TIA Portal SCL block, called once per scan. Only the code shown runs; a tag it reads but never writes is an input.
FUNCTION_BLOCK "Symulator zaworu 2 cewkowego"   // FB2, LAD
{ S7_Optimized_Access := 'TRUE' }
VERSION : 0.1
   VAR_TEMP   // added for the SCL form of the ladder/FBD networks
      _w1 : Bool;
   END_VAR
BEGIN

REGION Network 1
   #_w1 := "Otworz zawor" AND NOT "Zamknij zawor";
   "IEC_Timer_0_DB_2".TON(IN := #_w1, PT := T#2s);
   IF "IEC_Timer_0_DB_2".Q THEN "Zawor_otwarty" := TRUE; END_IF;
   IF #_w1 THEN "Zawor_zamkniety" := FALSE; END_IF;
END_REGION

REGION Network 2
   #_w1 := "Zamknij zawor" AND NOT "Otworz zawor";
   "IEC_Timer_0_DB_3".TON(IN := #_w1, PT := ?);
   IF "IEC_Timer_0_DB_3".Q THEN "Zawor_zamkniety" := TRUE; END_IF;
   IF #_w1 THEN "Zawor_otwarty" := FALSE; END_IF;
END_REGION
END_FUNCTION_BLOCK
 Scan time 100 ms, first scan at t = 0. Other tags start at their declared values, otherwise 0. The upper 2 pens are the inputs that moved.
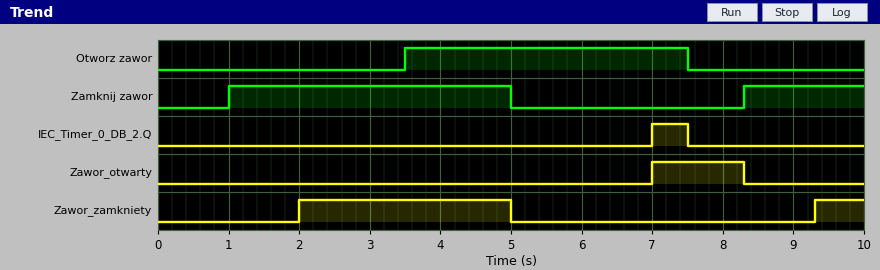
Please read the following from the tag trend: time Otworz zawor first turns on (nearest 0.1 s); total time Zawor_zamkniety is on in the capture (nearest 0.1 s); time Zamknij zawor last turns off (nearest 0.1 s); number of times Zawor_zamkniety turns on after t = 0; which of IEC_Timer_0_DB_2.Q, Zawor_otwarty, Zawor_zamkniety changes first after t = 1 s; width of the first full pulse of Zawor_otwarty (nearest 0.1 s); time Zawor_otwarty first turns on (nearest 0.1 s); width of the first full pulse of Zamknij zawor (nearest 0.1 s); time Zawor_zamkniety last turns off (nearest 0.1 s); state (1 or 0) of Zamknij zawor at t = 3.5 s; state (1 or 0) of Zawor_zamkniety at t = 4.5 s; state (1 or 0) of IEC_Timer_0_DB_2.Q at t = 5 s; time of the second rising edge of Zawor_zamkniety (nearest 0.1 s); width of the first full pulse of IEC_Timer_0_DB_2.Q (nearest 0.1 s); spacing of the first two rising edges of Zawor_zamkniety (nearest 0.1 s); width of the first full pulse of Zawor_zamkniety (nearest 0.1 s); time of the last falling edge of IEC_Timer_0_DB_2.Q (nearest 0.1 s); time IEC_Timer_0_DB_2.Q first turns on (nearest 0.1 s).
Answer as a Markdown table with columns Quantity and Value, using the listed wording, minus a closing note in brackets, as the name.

| Quantity | Value |
|---|---|
| time Otworz zawor first turns on | 3.5 s |
| total time Zawor_zamkniety is on in the capture | 3.7 s |
| time Zamknij zawor last turns off | 5.0 s |
| number of times Zawor_zamkniety turns on after t = 0 | 2 |
| which of IEC_Timer_0_DB_2.Q, Zawor_otwarty, Zawor_zamkniety changes first after t = 1 s | Zawor_zamkniety |
| width of the first full pulse of Zawor_otwarty | 1.3 s |
| time Zawor_otwarty first turns on | 7.0 s |
| width of the first full pulse of Zamknij zawor | 4.0 s |
| time Zawor_zamkniety last turns off | 5.0 s |
| state (1 or 0) of Zamknij zawor at t = 3.5 s | 1 |
| state (1 or 0) of Zawor_zamkniety at t = 4.5 s | 1 |
| state (1 or 0) of IEC_Timer_0_DB_2.Q at t = 5 s | 0 |
| time of the second rising edge of Zawor_zamkniety | 9.3 s |
| width of the first full pulse of IEC_Timer_0_DB_2.Q | 0.5 s |
| spacing of the first two rising edges of Zawor_zamkniety | 7.3 s |
| width of the first full pulse of Zawor_zamkniety | 3.0 s |
| time of the last falling edge of IEC_Timer_0_DB_2.Q | 7.5 s |
| time IEC_Timer_0_DB_2.Q first turns on | 7.0 s |
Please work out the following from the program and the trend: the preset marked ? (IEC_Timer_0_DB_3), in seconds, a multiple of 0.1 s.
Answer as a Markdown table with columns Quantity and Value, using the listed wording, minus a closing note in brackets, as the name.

| Quantity | Value |
|---|---|
| the preset marked ? (IEC_Timer_0_DB_3), in seconds, a multiple of 0.1 s | 1.0 s |
